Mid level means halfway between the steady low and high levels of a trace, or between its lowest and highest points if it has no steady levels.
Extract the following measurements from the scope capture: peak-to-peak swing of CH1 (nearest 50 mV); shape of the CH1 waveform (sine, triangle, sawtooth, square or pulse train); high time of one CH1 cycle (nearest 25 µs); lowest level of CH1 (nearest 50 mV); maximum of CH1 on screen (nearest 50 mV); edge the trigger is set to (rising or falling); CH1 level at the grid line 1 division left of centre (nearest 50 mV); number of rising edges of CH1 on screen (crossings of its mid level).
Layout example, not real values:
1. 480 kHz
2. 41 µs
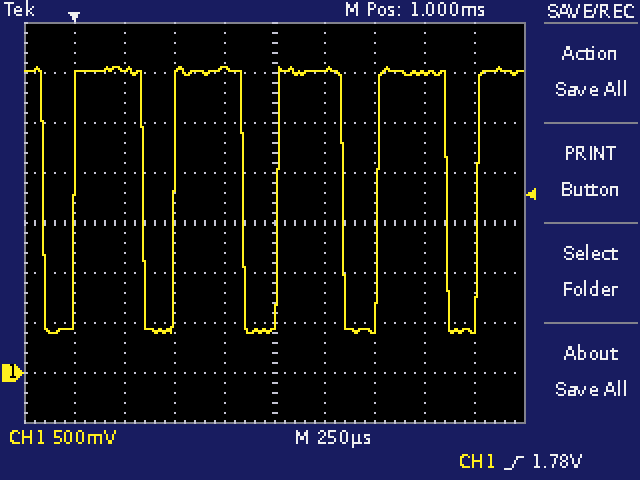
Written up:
1. 2.65 V
2. pulse train
3. 350 µs
4. 400 mV
5. 3.05 V
6. rising
7. 3.05 V
8. 5
